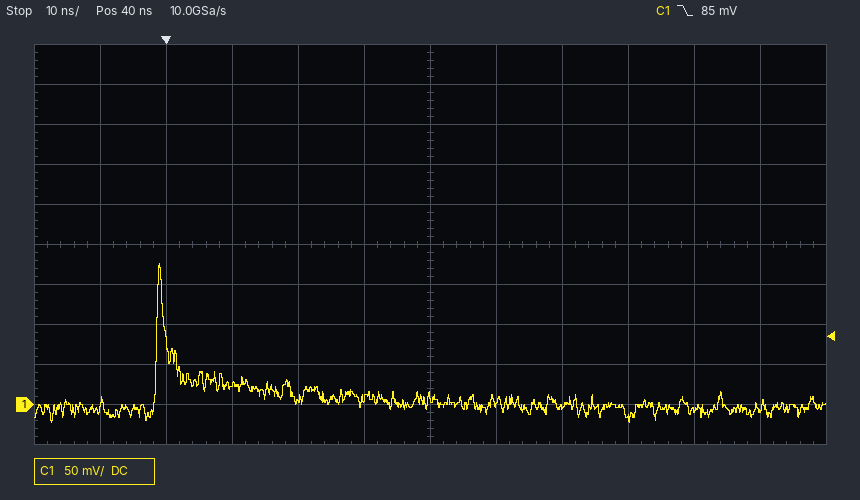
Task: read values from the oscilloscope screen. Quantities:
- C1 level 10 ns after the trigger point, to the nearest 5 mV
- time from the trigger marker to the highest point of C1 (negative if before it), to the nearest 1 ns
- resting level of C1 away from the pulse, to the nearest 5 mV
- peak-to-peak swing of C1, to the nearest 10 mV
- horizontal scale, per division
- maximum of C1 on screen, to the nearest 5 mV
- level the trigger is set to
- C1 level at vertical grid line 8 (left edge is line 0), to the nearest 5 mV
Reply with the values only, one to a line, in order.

25 mV
-1 ns
0 mV
200 mV
10 ns
175 mV
85 mV
0 mV
